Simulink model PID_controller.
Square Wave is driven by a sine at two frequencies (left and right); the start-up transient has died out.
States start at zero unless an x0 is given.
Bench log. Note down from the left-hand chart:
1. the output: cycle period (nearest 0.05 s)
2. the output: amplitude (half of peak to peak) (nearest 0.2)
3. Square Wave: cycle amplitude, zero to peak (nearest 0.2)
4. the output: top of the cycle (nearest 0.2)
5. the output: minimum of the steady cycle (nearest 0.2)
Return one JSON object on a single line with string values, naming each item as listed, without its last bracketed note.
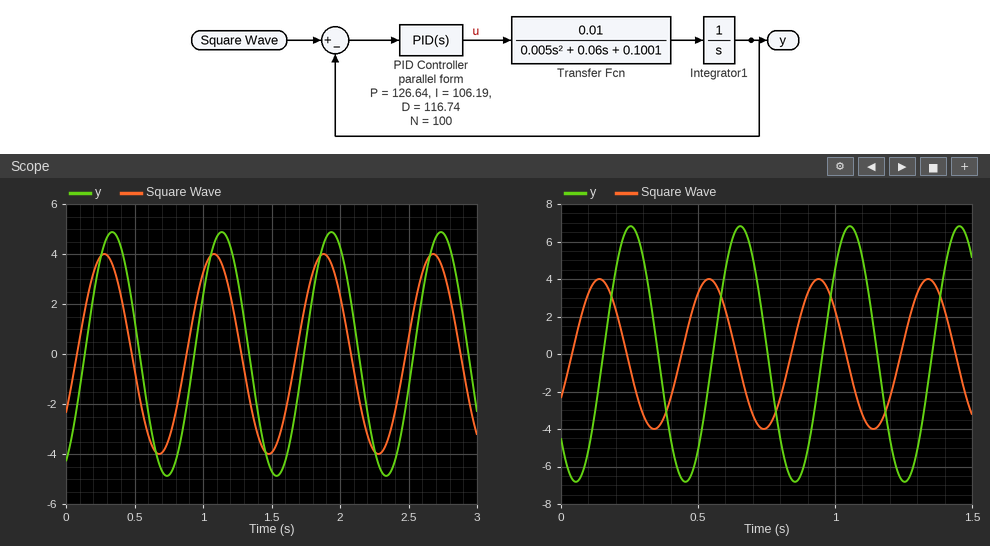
{"the output: cycle period": "0.80 s", "the output: amplitude (half of peak to peak)": "4.8", "Square Wave: cycle amplitude, zero to peak": "4.0", "the output: top of the cycle": "4.8", "the output: minimum of the steady cycle": "-4.8"}
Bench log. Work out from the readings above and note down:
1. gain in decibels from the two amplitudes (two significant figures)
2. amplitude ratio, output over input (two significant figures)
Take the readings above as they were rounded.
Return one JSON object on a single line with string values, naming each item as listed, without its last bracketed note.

{"gain in decibels from the two amplitudes": "1.6 dB", "amplitude ratio, output over input": "1.2"}
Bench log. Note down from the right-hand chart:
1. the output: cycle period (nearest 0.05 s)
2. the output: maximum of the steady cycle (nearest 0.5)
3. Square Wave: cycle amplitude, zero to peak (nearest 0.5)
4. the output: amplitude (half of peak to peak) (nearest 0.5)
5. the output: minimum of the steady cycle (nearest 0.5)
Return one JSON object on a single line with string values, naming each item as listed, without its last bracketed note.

{"the output: cycle period": "0.40 s", "the output: maximum of the steady cycle": "7.0", "Square Wave: cycle amplitude, zero to peak": "4.0", "the output: amplitude (half of peak to peak)": "7.0", "the output: minimum of the steady cycle": "-7.0"}
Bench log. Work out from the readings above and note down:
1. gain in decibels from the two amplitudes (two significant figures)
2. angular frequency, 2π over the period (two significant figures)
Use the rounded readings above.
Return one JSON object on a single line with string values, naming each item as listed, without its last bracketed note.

{"gain in decibels from the two amplitudes": "4.9 dB", "angular frequency, 2π over the period": "16 rad/s"}
